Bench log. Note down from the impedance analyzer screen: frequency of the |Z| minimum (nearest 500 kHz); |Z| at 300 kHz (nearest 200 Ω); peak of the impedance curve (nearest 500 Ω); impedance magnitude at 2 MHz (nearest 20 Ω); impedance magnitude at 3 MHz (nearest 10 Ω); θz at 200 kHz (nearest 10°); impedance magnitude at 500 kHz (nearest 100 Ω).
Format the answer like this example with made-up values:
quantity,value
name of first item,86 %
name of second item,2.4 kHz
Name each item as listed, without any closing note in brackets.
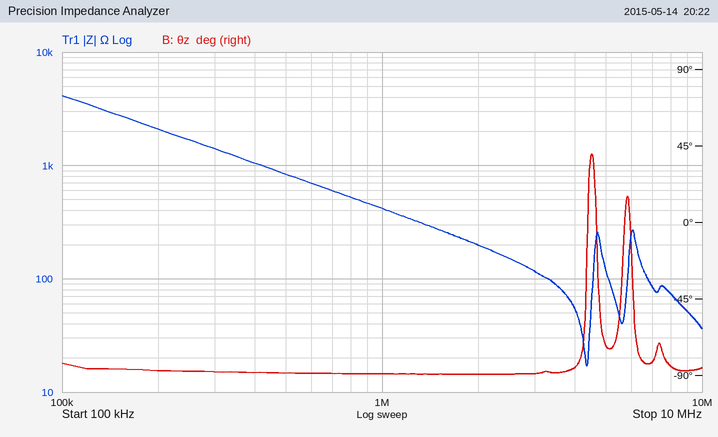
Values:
quantity,value
frequency of the |Z| minimum,4.5 MHz
|Z| at 300 kHz,1.4 kΩ
peak of the impedance curve,4.0 kΩ
impedance magnitude at 2 MHz,200 Ω
impedance magnitude at 3 MHz,120 Ω
θz at 200 kHz,-90°
impedance magnitude at 500 kHz,800 Ω
